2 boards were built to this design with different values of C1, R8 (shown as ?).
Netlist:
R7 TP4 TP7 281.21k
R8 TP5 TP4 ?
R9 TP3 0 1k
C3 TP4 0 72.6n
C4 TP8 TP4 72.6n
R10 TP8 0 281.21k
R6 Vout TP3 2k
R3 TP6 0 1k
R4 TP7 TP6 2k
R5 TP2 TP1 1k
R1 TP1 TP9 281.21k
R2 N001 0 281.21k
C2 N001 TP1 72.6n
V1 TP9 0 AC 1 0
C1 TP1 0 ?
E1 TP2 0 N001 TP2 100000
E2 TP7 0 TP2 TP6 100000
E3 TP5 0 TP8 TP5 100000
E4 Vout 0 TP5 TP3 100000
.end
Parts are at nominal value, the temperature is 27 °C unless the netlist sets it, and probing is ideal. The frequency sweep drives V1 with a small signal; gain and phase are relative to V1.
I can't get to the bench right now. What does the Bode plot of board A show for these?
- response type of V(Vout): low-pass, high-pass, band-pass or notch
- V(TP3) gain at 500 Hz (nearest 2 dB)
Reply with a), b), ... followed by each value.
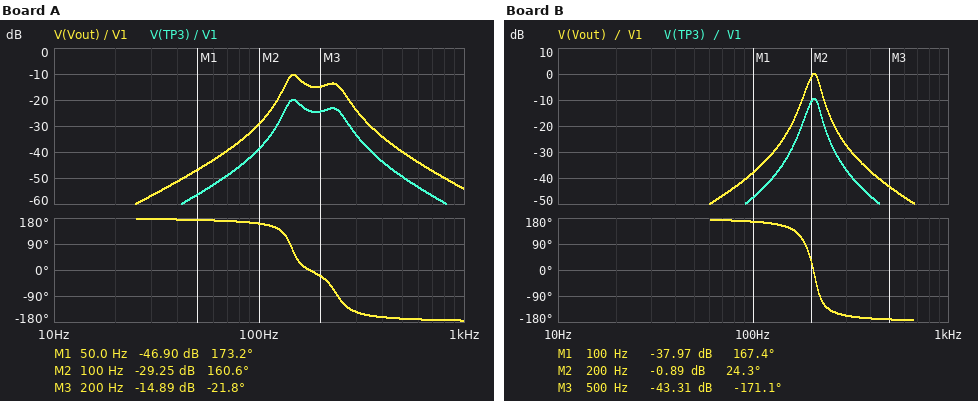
a) band-pass
b) -50 dB
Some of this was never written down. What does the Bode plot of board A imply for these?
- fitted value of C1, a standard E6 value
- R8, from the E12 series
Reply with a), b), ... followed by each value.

a) 22 nF
b) 820 Ω
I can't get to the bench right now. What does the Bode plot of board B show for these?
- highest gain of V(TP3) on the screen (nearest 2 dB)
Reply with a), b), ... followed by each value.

a) -10 dB
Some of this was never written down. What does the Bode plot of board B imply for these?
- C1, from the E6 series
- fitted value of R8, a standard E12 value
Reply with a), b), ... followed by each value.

a) 33 nF
b) 390 Ω
